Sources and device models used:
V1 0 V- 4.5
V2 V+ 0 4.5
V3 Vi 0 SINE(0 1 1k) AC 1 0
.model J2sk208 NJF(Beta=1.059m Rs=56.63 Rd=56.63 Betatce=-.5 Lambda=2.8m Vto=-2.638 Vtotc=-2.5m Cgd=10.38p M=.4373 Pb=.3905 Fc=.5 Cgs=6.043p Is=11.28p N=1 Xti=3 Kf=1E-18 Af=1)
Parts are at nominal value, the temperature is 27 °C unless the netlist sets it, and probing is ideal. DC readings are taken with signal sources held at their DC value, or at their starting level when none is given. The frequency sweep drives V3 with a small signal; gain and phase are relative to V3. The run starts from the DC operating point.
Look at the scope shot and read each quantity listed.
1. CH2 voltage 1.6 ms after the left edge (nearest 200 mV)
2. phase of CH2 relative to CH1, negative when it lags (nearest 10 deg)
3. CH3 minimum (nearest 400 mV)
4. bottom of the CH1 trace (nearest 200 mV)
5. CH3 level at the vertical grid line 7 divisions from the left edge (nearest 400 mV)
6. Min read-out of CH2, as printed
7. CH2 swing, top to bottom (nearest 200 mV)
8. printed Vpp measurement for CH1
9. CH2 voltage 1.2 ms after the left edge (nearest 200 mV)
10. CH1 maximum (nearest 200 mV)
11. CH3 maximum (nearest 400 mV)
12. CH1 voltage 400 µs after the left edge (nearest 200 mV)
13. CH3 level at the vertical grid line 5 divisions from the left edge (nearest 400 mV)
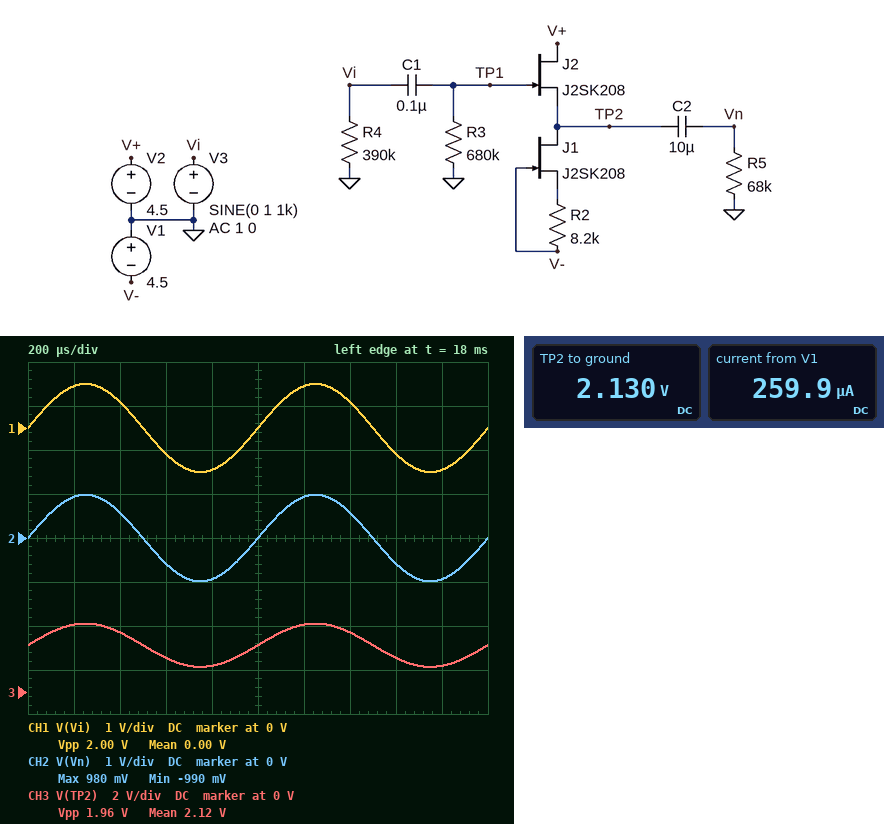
-600 mV
0 deg
1.2 V
-1.0 V
2.8 V
-990 mV
2.0 V
2.00 V
1.0 V
1.0 V
3.2 V
600 mV
2.0 V
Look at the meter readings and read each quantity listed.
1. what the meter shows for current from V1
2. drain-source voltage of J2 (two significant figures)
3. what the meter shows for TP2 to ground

259.9 µA
2.4 V
2.130 V
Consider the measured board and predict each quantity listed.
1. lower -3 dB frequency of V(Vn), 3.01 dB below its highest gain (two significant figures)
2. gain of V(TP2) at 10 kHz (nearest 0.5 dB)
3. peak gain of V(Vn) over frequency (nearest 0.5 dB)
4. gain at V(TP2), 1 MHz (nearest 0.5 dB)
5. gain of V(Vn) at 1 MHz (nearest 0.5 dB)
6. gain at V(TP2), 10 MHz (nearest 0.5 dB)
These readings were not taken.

2.4 Hz
0 dB
0 dB
0 dB
0 dB
-0.5 dB
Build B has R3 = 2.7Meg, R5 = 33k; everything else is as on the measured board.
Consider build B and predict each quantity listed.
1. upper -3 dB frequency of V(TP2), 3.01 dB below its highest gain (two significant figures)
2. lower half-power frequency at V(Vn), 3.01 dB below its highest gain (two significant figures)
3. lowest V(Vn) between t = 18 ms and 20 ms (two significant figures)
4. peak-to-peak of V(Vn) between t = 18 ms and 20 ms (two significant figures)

48 MHz
820 mHz
-970 mV
1.9 V
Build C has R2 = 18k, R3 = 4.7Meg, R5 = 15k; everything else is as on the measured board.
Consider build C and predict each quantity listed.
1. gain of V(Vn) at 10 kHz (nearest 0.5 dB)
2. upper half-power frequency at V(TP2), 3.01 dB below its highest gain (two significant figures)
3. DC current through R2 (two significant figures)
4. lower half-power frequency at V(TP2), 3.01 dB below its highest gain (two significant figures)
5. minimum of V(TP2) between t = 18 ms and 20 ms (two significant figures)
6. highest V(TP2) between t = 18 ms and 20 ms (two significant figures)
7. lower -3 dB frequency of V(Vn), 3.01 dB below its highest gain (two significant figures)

-1.0 dB
39 MHz
130 µA
290 mHz
1.4 V
3.2 V
1.1 Hz
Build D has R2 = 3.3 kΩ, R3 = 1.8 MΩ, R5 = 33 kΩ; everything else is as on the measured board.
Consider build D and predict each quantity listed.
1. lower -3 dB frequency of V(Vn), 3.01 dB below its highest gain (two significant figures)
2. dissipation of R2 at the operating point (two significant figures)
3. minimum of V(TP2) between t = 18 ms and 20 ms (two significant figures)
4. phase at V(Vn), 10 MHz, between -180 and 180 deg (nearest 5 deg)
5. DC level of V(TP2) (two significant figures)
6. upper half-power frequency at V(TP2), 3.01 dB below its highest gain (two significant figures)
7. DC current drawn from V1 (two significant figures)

1.1 Hz
1.1 mW
900 mV
-5 deg
1.9 V
67 MHz
570 µA
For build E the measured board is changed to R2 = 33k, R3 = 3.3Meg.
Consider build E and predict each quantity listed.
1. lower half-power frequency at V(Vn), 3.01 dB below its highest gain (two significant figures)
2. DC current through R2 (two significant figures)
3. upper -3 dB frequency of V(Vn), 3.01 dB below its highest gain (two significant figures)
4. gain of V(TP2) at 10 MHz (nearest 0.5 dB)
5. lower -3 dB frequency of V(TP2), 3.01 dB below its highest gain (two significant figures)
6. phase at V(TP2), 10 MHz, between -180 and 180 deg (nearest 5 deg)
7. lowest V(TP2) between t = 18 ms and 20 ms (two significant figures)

570 mHz
72 µA
26 MHz
-1.0 dB
480 mHz
-15 deg
1.4 V
